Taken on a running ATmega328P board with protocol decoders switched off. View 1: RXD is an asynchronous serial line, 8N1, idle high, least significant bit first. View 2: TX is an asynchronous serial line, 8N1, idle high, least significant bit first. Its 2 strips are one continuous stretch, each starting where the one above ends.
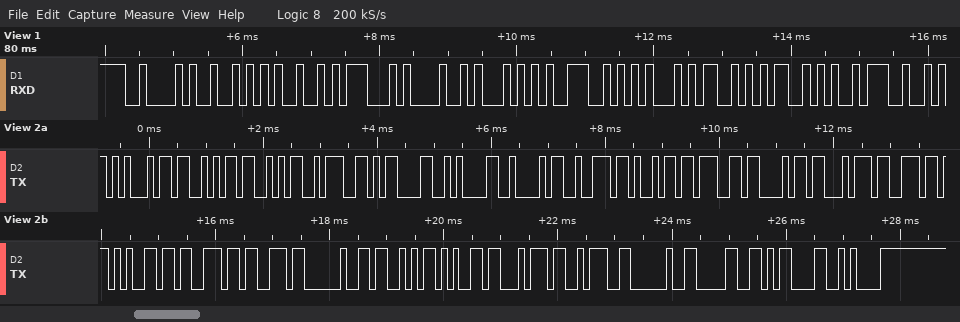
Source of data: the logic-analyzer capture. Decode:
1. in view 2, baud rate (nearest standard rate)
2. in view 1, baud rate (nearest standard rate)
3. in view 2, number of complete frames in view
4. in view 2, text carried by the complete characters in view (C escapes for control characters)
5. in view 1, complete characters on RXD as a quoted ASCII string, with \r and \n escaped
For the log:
9600 baud
9600 baud
25
"ESS:\r\nBrightness Set: 0\r\n"
"BRIGHTNESS:"
